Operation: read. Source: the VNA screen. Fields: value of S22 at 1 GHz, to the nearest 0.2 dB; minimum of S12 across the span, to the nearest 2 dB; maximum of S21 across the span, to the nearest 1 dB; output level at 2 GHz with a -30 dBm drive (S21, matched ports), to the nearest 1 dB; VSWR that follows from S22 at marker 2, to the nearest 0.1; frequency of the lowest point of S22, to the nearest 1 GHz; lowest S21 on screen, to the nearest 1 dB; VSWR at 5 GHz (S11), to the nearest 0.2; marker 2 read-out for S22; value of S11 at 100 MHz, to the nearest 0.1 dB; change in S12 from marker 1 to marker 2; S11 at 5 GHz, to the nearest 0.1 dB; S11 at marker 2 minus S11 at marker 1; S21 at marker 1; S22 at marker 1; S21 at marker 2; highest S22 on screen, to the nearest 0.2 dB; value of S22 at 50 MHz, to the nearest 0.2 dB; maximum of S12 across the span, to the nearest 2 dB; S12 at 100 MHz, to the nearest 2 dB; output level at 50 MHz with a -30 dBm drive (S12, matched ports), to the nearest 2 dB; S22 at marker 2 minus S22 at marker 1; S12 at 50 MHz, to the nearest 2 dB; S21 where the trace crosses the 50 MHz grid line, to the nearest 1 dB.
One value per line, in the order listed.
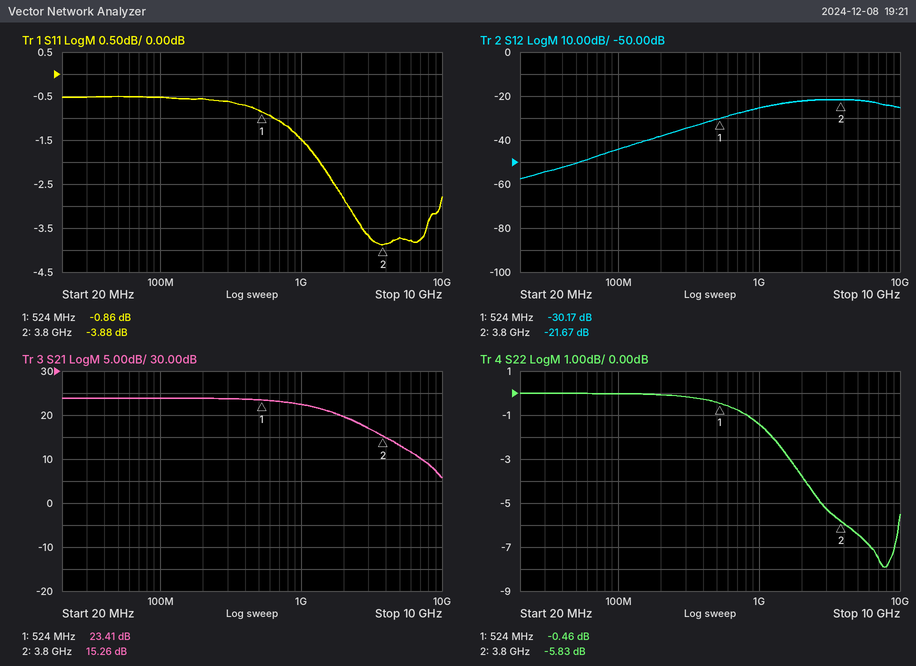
-1.4 dB
-58 dB
24 dB
-10 dBm
3.1
8 GHz
6 dB
4.8
-5.83 dB
-0.5 dB
8.50 dB
-3.7 dB
-3.02 dB
23.41 dB
-0.46 dB
15.26 dB
0.0 dB
0.0 dB
-22 dB
-44 dB
-80 dBm
-5.37 dB
-50 dB
24 dB
